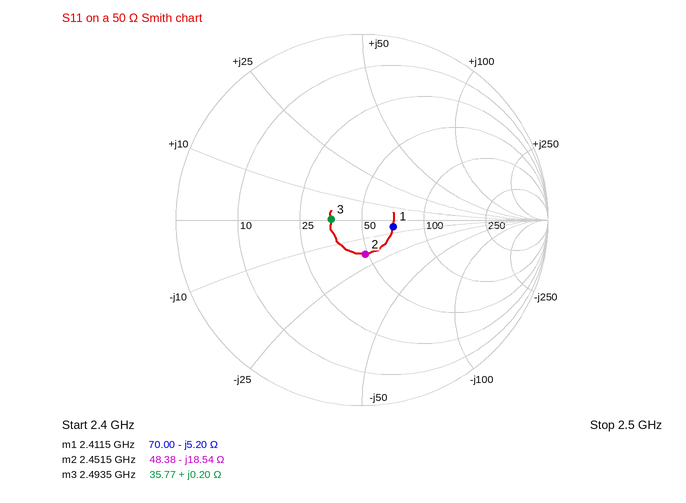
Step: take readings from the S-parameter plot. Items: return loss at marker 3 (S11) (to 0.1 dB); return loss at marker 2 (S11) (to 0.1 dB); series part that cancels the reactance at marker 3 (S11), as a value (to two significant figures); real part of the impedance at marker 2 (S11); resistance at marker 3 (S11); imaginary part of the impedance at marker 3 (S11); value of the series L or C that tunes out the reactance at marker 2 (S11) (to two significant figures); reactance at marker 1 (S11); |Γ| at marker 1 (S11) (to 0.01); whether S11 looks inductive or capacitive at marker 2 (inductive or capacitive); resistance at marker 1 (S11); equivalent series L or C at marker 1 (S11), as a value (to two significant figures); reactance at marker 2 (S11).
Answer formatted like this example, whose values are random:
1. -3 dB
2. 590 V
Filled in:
1. 15.6 dB
2. 14.6 dB
3. 320 pF
4. 48.38 Ω
5. 35.77 Ω
6. +0.20 Ω
7. 1.2 nH
8. -5.20 Ω
9. 0.17
10. capacitive
11. 70.00 Ω
12. 13 pF
13. -18.54 Ω
